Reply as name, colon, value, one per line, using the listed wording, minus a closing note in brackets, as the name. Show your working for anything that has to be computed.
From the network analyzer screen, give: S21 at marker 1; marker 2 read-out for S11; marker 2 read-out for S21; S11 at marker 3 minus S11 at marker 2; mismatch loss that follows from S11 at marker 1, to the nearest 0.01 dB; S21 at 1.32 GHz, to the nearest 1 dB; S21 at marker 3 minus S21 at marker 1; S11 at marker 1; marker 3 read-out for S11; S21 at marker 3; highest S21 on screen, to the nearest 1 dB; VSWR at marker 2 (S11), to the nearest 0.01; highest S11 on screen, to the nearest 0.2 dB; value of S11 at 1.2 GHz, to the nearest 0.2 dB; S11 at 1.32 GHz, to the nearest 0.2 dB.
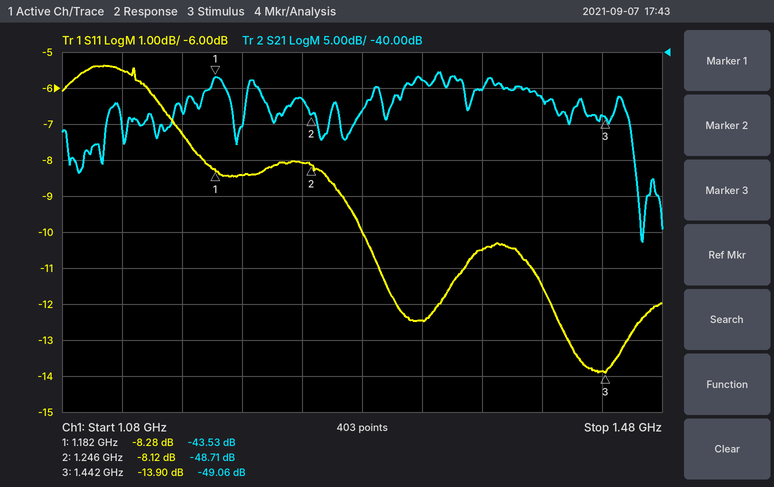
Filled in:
S21 at marker 1: -43.53 dB
marker 2 read-out for S11: -8.12 dB
marker 2 read-out for S21: -48.71 dB
S11 at marker 3 minus S11 at marker 2: -13.9 − (-8.12) = -5.78 dB
mismatch loss that follows from S11 at marker 1, to the nearest 0.01 dB: −10 log10(1 − 10^(-8.28/10)) ≈ 0.70 dB
S21 at 1.32 GHz, to the nearest 1 dB: -44 dB
S21 at marker 3 minus S21 at marker 1: -49.06 − (-43.53) = -5.53 dB
S11 at marker 1: -8.28 dB
marker 3 read-out for S11: -13.90 dB
S21 at marker 3: -49.06 dB
highest S21 on screen, to the nearest 1 dB: -43 dB
VSWR at marker 2 (S11), to the nearest 0.01: (1 + 0.3926)/(1 − 0.3926) ≈ 2.29
highest S11 on screen, to the nearest 0.2 dB: -5.4 dB
value of S11 at 1.2 GHz, to the nearest 0.2 dB: -8.4 dB
S11 at 1.32 GHz, to the nearest 0.2 dB: -12.4 dB
